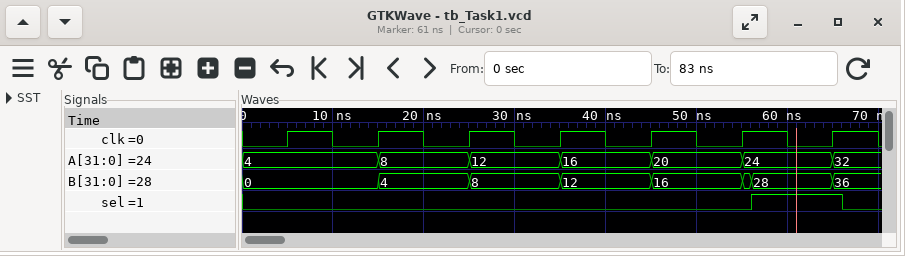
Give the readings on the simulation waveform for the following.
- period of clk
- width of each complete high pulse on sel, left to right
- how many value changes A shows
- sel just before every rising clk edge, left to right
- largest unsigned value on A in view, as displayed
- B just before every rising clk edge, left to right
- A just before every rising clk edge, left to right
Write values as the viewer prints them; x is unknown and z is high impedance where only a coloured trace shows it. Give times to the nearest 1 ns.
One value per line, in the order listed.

10 ns
10 ns
6
0 0 0 0 0 0 1
32
0, 0, 4, 8, 12, 16, 28
4, 4, 8, 12, 16, 20, 24
